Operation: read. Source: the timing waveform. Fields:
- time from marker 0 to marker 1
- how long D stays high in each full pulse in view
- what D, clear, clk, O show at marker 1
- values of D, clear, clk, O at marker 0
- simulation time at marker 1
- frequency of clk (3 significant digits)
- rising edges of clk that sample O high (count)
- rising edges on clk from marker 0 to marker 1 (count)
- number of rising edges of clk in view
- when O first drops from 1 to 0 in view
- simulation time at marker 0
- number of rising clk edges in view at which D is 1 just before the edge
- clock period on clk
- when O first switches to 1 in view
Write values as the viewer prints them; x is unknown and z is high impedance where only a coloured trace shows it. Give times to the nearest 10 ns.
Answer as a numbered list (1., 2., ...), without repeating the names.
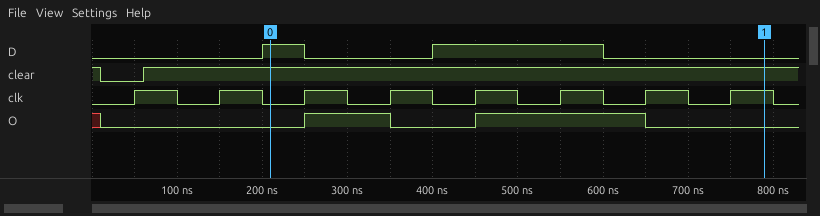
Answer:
1. 580 ns
2. 50 ns, 200 ns
3. D=0, clear=1, clk=1, O=0
4. D=1, clear=1, clk=0, O=0
5. 790 ns
6. 10.0 MHz
7. 3
8. 6
9. 8
10. 350 ns
11. 210 ns
12. 3
13. 100 ns
14. 250 ns
